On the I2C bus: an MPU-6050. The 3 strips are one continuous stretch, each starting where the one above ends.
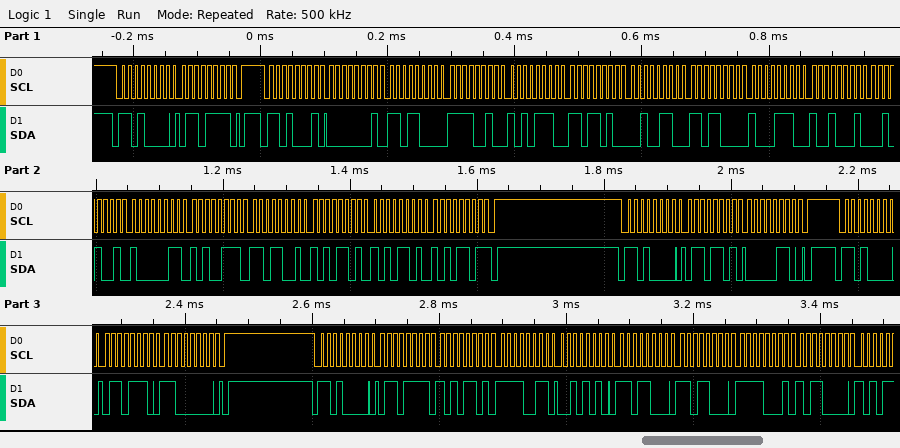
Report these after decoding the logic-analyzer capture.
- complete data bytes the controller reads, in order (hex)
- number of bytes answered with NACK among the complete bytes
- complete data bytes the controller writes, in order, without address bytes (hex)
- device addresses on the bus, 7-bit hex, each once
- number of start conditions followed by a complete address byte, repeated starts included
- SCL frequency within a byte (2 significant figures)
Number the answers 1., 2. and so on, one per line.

1. 01 D8 F2 AE DA 26 D8 8E 91 29 83 A7 D9 AD AD AD
2. 1
3. 6F 6D 06 6E C0 6F AD F3 2A D8 D8 F1 B0
4. 0x68
5. 5
6. 100 kHz
